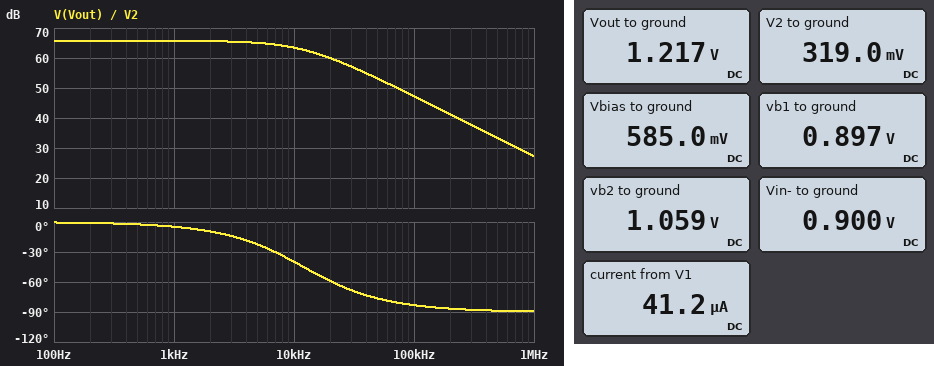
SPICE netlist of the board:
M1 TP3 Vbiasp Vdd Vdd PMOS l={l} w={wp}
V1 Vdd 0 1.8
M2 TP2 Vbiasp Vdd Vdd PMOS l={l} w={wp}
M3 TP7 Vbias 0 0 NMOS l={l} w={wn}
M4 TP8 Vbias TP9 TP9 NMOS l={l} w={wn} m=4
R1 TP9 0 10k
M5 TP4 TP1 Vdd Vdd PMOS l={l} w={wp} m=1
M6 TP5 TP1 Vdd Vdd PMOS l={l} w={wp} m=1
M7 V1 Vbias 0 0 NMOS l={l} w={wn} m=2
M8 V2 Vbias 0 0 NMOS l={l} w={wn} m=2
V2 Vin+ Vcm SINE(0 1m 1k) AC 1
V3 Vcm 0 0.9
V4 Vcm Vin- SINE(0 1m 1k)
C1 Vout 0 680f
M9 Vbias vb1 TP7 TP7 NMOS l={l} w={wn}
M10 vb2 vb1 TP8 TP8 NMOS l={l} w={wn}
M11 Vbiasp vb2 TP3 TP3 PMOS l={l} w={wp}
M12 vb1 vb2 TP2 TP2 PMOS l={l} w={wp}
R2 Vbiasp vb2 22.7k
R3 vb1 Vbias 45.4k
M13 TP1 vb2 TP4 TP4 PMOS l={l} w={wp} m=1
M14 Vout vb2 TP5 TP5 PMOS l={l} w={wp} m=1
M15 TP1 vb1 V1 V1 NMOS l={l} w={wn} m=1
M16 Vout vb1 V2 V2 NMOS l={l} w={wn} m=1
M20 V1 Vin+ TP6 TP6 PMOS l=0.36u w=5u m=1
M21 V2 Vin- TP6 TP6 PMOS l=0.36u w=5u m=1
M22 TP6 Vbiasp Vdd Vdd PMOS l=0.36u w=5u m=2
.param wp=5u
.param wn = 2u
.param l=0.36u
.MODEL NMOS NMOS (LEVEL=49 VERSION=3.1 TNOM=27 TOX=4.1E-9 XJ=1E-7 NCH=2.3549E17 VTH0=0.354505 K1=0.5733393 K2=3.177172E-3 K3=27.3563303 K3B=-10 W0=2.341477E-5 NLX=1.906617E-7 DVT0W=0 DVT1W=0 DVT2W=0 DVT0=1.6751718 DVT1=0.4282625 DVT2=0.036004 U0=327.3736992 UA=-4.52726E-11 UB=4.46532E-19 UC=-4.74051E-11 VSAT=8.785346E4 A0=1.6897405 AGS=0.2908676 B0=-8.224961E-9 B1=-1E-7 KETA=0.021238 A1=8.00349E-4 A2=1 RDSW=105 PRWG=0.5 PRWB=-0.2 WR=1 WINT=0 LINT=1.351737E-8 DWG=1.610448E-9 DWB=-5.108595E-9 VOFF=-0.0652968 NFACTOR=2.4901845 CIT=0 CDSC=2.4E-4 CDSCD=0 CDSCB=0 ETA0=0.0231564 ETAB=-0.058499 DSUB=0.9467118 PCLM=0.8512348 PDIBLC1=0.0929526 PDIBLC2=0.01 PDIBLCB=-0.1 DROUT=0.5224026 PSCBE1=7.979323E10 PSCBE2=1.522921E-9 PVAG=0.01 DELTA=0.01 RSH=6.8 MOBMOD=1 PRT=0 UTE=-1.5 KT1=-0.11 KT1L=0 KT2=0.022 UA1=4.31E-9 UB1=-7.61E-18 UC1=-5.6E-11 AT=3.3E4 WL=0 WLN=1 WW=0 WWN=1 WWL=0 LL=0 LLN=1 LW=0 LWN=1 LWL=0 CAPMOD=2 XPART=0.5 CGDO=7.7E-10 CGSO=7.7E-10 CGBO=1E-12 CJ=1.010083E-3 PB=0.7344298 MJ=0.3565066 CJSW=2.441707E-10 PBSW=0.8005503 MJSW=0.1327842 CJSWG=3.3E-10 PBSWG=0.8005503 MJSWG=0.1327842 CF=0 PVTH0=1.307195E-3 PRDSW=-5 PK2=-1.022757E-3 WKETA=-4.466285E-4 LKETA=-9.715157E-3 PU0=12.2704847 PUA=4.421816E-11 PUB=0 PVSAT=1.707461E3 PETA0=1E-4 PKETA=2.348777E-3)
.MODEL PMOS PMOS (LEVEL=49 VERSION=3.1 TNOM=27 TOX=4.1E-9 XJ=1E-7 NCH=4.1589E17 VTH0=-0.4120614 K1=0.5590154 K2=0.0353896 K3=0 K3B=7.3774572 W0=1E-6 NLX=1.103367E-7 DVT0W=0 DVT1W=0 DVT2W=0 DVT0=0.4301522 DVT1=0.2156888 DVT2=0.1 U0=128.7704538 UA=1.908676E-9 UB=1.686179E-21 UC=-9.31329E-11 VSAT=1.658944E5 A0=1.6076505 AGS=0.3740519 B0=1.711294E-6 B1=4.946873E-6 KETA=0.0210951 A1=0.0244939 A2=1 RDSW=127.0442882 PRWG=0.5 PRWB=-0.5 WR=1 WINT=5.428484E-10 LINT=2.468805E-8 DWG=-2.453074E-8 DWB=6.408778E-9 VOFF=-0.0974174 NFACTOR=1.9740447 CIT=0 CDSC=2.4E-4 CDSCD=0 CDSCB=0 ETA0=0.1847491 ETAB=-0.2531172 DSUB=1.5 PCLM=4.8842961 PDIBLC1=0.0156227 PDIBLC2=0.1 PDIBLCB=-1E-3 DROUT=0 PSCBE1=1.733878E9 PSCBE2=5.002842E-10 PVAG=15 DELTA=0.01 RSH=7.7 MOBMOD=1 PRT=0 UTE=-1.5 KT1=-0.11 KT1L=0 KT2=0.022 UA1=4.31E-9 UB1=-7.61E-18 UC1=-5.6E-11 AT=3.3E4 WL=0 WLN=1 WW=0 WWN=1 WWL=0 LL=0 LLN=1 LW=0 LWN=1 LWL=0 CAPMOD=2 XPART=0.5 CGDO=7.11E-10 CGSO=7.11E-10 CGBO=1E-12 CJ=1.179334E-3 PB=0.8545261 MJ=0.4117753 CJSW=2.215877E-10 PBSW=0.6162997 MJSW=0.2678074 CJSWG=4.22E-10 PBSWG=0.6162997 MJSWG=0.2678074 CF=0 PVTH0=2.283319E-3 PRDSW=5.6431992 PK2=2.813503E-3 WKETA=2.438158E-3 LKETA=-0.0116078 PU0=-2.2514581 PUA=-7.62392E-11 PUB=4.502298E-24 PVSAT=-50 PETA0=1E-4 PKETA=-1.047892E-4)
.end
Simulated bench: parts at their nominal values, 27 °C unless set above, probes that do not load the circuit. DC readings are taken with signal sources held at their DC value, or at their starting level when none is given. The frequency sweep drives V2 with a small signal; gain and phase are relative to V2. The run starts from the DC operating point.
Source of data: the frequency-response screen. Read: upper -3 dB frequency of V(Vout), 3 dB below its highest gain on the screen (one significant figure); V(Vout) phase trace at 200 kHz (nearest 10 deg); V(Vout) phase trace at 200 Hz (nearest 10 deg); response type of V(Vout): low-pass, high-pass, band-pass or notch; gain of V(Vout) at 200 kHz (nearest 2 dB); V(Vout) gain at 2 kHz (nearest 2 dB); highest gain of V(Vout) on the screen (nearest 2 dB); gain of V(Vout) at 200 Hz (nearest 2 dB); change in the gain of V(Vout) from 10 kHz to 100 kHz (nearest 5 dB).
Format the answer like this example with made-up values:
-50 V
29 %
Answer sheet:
10 kHz
-90 deg
0 deg
low-pass
42 dB
66 dB
66 dB
66 dB
-15 dB
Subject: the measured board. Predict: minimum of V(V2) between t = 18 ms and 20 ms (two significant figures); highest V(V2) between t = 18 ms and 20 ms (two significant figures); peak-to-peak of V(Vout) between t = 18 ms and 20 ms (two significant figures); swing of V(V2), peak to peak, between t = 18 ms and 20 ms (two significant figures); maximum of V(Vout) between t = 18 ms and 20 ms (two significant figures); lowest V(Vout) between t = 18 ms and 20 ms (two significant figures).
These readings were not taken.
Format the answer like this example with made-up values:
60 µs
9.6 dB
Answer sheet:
270 mV
320 mV
1.3 V
54 mV
1.6 V
310 mV
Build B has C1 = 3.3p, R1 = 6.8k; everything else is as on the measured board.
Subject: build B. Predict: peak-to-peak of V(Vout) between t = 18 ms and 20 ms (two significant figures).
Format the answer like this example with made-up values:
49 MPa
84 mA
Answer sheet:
1.1 V
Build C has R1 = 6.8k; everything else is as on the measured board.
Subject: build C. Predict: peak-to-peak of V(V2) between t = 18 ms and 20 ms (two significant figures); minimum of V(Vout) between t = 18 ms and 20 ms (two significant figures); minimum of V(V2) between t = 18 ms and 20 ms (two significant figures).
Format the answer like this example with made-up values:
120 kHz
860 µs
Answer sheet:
62 mV
500 mV
450 mV
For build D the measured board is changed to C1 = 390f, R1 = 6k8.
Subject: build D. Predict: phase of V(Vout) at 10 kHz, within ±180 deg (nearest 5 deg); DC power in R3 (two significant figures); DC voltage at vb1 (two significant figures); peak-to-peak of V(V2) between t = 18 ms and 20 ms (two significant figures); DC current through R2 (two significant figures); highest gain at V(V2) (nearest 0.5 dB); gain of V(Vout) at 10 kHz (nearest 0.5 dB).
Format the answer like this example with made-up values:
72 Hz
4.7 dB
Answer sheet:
-25 deg
5.6 µW
1.1 V
62 mV
11 µA
26.5 dB
67.0 dB
